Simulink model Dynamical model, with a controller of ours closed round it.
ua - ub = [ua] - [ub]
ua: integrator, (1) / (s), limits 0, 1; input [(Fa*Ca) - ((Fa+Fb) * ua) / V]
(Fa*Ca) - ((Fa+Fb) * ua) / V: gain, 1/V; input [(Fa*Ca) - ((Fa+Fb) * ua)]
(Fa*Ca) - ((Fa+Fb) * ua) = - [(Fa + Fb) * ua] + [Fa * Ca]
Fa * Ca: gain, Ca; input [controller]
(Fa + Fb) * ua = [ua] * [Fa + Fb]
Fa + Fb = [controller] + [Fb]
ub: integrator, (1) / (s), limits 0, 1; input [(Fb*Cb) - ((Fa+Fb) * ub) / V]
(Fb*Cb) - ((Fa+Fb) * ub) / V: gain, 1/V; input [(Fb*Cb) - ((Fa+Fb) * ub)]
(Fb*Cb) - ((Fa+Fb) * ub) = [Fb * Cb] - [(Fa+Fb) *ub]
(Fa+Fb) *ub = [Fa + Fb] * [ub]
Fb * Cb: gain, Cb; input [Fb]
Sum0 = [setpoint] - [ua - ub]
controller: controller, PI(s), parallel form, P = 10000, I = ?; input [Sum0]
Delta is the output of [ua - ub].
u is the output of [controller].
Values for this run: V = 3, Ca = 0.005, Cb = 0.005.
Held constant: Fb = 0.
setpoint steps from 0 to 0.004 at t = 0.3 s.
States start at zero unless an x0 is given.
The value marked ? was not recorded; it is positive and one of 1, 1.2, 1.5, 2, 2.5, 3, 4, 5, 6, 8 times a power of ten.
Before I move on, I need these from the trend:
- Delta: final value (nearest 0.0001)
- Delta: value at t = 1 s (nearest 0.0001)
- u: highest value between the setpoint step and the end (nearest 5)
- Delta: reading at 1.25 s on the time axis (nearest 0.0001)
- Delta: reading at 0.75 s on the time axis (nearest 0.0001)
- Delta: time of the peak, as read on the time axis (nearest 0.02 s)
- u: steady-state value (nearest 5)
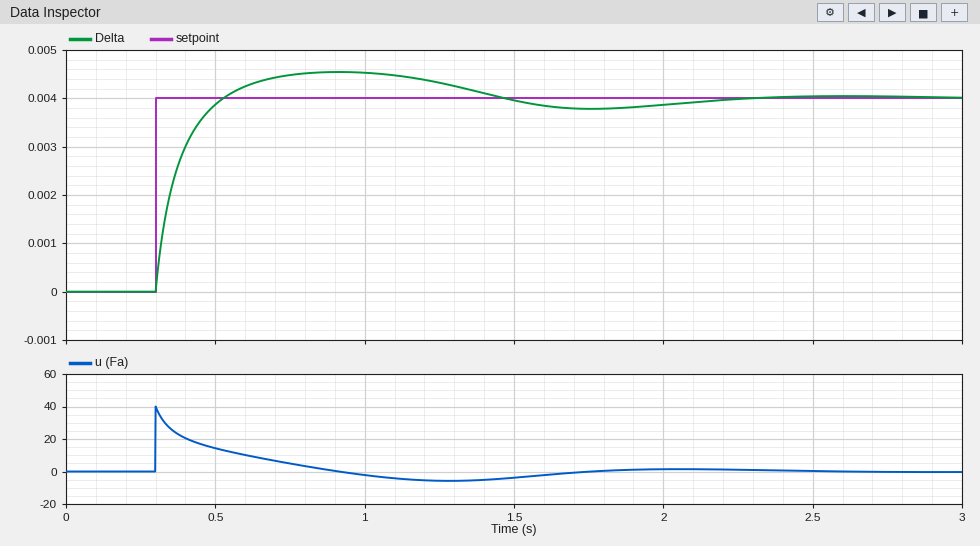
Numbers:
0.0040
0.0045
40
0.0043
0.0045
0.92 s
0
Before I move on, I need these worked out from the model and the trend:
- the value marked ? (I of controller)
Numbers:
50000
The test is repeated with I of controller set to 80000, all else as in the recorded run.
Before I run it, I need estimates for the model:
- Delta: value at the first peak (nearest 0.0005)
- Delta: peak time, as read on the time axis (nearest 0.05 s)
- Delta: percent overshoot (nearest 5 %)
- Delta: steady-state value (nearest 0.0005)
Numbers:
0.0045
0.80 s
15 %
0.0040
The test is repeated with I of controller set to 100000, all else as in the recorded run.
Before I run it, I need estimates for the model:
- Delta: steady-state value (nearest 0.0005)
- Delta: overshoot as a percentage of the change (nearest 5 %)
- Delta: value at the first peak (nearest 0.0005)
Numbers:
0.0040
15 %
0.0045
